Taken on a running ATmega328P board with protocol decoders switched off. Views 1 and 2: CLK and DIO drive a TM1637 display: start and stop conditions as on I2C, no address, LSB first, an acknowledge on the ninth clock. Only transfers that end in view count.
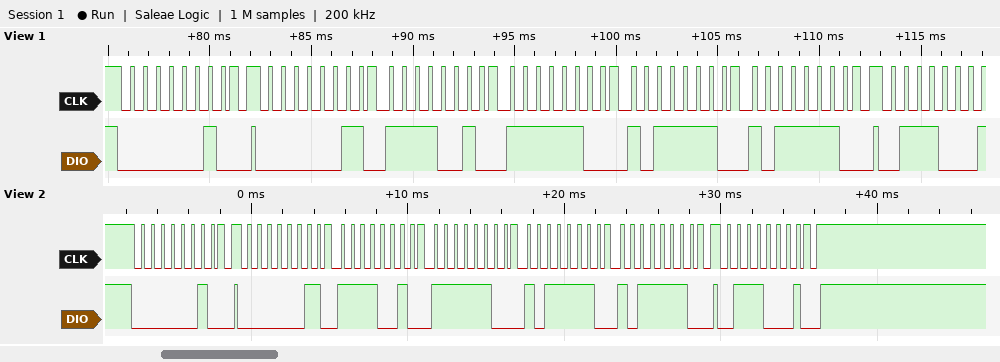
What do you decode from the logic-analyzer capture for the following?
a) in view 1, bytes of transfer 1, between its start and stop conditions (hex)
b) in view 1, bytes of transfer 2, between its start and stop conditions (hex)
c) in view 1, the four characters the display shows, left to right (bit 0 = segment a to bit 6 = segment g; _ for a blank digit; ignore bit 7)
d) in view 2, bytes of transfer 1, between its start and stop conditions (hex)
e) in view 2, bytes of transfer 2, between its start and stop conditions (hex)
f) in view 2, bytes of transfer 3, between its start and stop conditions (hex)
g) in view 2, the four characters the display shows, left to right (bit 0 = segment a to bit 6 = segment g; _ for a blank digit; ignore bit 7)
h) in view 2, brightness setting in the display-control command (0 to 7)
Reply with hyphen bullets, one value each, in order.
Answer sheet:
- 40
- C0 4F 3F 7D 7D
- 3066
- 40
- C0 4F 3F 7D 7D
- 8E
- 3066
- 6
